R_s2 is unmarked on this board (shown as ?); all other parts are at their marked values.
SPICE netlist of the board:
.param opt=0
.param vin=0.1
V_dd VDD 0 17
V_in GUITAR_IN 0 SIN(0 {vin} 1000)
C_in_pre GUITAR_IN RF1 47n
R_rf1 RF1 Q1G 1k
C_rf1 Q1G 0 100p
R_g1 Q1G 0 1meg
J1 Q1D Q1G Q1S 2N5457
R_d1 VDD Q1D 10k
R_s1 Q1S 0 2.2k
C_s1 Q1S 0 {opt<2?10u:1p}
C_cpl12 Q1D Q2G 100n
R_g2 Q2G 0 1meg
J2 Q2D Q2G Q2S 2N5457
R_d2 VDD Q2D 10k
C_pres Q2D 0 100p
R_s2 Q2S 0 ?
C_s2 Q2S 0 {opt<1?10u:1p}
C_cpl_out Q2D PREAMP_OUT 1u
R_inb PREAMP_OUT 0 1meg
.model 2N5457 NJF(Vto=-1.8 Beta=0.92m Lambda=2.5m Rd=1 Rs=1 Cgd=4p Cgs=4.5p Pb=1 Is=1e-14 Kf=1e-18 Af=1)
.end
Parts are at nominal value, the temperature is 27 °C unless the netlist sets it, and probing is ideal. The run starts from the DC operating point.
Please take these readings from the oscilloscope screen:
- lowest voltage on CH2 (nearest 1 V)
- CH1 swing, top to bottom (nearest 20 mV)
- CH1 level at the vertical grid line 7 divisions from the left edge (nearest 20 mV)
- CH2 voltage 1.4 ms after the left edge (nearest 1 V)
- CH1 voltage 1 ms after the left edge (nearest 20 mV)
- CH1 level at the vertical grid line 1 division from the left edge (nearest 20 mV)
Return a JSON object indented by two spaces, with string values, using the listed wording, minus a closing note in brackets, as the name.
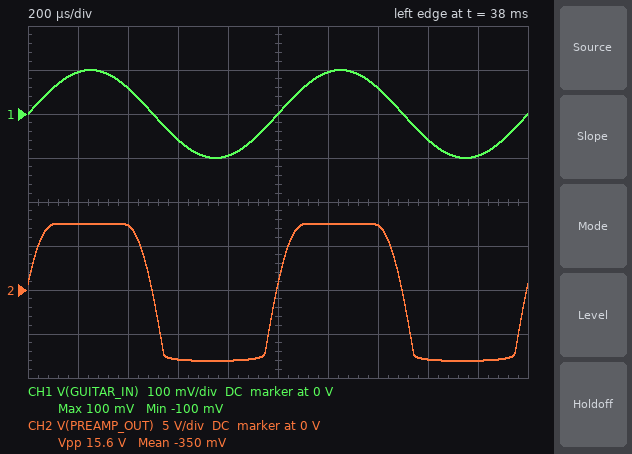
{
  "lowest voltage on CH2": "-8 V",
  "CH1 swing, top to bottom": "200 mV",
  "CH1 level at the vertical grid line 7 divisions from the left edge": "60 mV",
  "CH2 voltage 1.4 ms after the left edge": "7 V",
  "CH1 voltage 1 ms after the left edge": "0 V",
  "CH1 level at the vertical grid line 1 division from the left edge": "100 mV"
}
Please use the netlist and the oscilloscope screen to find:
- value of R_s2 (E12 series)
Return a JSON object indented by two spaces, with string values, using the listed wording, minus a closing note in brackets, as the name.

{
  "value of R_s2": "1.2 kΩ"
}
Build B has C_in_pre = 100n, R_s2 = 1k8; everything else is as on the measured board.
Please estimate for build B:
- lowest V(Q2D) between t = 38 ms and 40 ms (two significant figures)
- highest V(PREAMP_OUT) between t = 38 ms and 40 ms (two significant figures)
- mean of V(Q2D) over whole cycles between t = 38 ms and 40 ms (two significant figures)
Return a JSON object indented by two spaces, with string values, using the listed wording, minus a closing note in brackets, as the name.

{
  "lowest V(Q2D) between t = 38 ms and 40 ms": "1.7 V",
  "highest V(PREAMP_OUT) between t = 38 ms and 40 ms": "5.7 V",
  "mean of V(Q2D) over whole cycles between t = 38 ms and 40 ms": "10 V"
}
